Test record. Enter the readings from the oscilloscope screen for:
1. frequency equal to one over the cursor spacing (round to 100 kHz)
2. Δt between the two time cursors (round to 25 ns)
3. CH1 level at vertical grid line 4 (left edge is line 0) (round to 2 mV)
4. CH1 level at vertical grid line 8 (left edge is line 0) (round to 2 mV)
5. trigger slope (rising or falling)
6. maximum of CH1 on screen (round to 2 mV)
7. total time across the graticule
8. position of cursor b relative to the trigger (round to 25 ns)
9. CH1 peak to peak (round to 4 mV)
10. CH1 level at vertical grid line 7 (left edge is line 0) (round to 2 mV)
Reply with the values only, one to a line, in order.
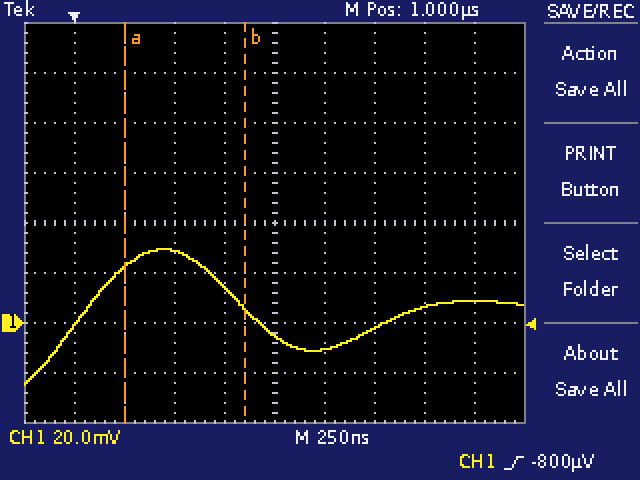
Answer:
1.7 MHz
600 ns
14 mV
6 mV
rising
30 mV
2.5 µs
+850 ns
56 mV
-2 mV
